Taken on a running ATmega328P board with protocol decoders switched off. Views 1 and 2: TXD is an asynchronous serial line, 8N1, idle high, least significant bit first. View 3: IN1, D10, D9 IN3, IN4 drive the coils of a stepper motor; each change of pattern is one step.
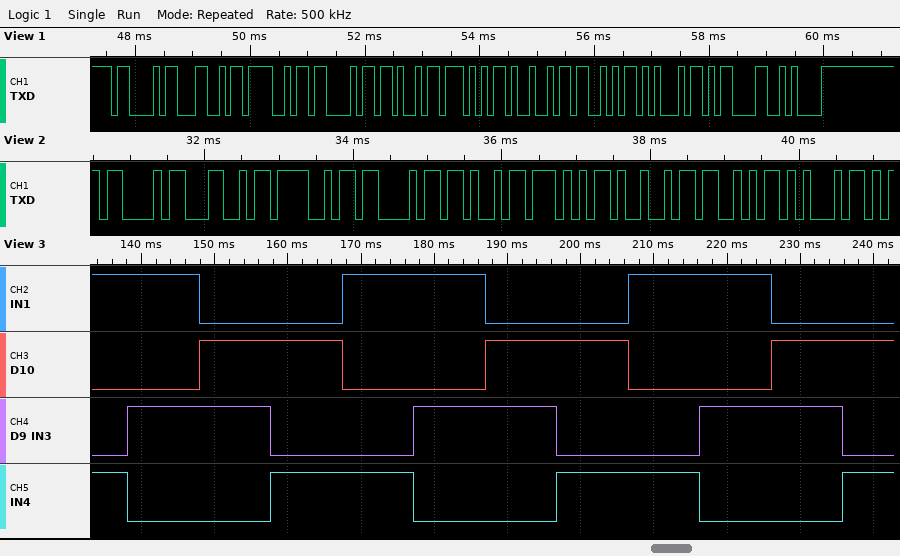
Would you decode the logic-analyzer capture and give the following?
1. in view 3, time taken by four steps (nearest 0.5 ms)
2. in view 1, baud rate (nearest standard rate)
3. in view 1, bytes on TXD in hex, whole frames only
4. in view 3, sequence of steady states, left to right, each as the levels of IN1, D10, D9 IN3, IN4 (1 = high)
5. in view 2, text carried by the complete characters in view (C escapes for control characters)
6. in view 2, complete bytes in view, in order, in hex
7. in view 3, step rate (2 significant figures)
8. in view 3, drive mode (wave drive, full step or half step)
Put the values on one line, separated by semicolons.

39.0 ms; 9600 baud; 43 4C 4F 43 4B 57 49 53 45 0D 0A; 1001 1010 0110 0101 1001 1010 0110 0101 1001 1010 0110 0101; "CLOCKWISE"; 43 4C 4F 43 4B 57 49 53 45; 100 steps/s; full step
